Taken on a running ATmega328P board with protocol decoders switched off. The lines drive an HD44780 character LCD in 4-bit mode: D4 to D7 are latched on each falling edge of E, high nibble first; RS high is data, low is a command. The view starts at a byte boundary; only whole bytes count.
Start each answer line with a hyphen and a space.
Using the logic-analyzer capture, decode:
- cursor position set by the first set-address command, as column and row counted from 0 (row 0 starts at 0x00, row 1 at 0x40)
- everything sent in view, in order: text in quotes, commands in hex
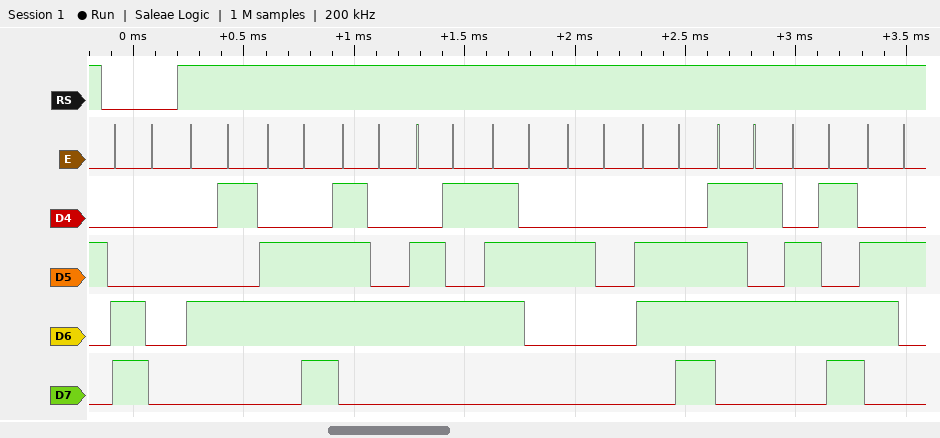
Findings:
- column 0, row 1
- 0xC0 "Enter numb"
